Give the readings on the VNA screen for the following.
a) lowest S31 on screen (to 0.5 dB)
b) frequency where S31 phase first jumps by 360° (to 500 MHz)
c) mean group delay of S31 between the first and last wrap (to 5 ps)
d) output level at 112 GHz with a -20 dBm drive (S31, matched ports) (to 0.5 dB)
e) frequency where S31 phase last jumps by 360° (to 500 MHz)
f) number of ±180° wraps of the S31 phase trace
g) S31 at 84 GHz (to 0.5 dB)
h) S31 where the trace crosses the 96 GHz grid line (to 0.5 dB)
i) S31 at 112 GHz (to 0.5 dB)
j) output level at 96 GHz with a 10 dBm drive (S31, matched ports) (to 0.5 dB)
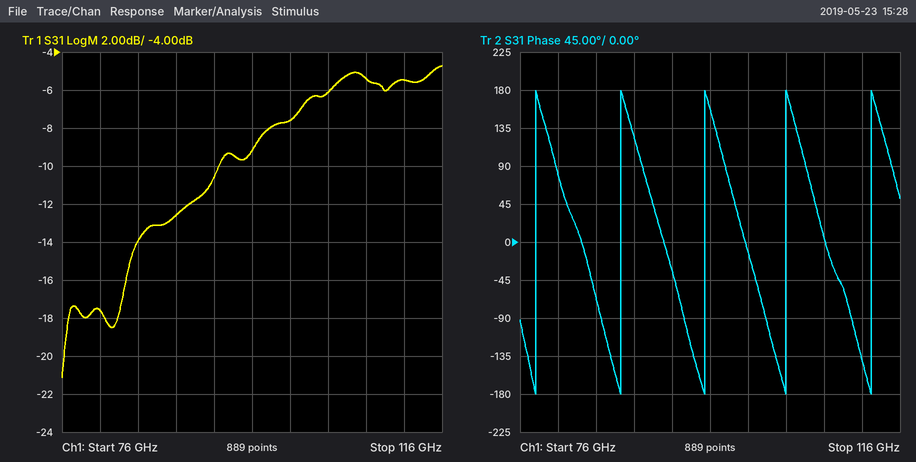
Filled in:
-21.0 dB
77.5 GHz
115 ps
-25.5 dBm
113.0 GHz
5
-14.0 dB
-9.0 dB
-5.5 dB
1.0 dBm
